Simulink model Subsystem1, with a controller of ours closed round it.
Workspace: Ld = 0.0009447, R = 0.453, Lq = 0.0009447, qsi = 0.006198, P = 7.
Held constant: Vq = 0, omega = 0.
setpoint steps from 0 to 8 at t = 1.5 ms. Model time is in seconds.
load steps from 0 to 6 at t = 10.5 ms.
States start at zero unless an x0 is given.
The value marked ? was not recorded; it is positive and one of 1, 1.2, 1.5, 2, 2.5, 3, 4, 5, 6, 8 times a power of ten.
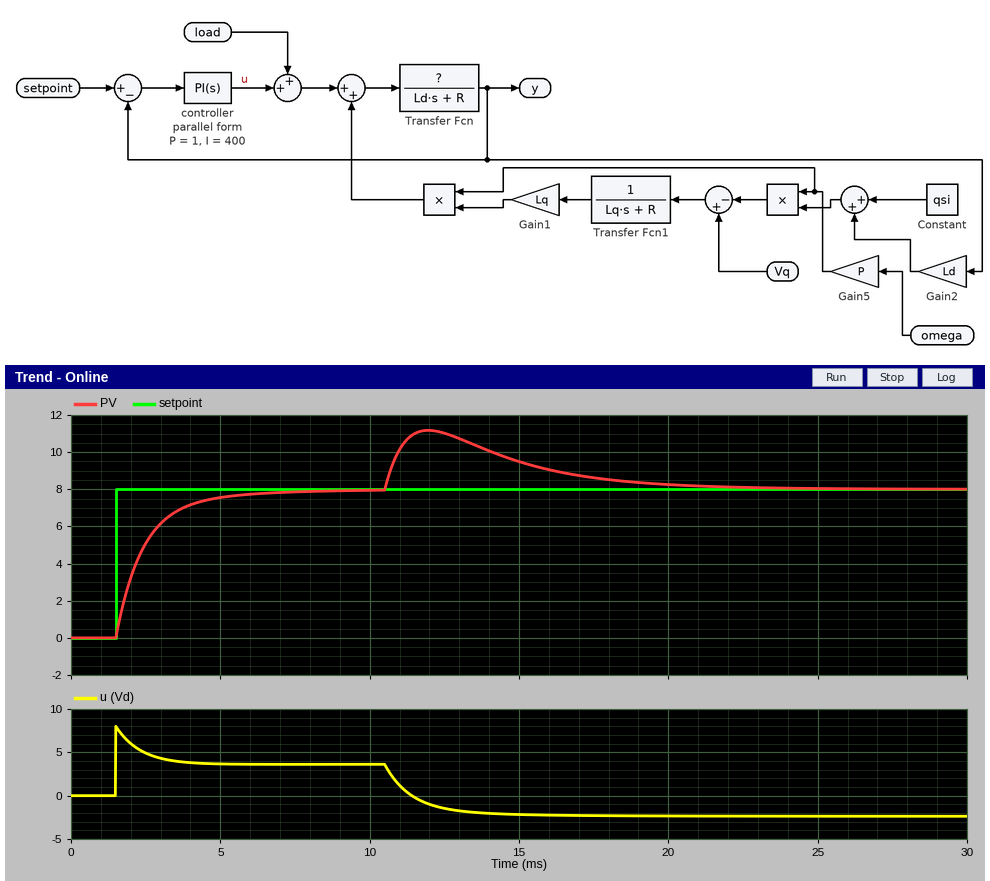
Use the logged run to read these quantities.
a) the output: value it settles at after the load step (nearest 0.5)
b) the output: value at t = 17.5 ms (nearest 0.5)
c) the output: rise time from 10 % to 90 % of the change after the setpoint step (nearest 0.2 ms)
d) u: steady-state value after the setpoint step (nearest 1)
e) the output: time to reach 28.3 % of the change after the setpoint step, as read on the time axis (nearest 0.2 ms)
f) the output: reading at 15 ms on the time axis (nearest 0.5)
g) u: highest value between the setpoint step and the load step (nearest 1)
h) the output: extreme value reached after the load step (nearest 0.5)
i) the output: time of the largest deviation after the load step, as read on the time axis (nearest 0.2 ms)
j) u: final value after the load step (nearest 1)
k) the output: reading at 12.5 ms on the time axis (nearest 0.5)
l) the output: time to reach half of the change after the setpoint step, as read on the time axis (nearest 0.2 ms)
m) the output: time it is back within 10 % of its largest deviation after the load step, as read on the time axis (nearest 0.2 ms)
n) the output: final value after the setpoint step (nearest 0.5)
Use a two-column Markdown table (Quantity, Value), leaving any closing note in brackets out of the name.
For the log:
| Quantity | Value |
|---|---|
| the output: value it settles at after the load step | 8.0 |
| the output: value at t = 17.5 ms | 8.5 |
| the output: rise time from 10 % to 90 % of the change after the setpoint step | 2.4 ms |
| u: steady-state value after the setpoint step | 4 |
| the output: time to reach 28.3 % of the change after the setpoint step, as read on the time axis | 1.8 ms |
| the output: reading at 15 ms on the time axis | 9.5 |
| u: highest value between the setpoint step and the load step | 8 |
| the output: extreme value reached after the load step | 11.0 |
| the output: time of the largest deviation after the load step, as read on the time axis | 12.0 ms |
| u: final value after the load step | -2 |
| the output: reading at 12.5 ms on the time axis | 11.0 |
| the output: time to reach half of the change after the setpoint step, as read on the time axis | 2.2 ms |
| the output: time it is back within 10 % of its largest deviation after the load step, as read on the time axis | 19.4 ms |
| the output: final value after the setpoint step | 8.0 |
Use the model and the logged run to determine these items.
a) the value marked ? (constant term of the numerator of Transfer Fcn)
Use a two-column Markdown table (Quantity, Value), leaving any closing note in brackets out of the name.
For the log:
| Quantity | Value |
|---|---|
| the value marked ? | 1 |
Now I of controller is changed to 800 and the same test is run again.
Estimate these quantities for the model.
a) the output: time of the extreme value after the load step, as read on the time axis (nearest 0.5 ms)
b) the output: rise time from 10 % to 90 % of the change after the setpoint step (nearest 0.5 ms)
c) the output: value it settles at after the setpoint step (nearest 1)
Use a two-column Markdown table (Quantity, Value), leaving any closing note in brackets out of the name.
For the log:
| Quantity | Value |
|---|---|
| the output: time of the extreme value after the load step, as read on the time axis | 11.5 ms |
| the output: rise time from 10 % to 90 % of the change after the setpoint step | 1.5 ms |
| the output: value it settles at after the setpoint step | 8 |
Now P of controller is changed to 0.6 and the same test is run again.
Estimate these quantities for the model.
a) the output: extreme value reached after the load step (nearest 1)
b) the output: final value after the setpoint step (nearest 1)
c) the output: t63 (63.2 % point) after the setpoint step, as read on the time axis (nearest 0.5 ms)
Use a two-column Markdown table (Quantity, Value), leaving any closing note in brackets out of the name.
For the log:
| Quantity | Value |
|---|---|
| the output: extreme value reached after the load step | 12 |
| the output: final value after the setpoint step | 8 |
| the output: t63 (63.2 % point) after the setpoint step, as read on the time axis | 3.0 ms |
